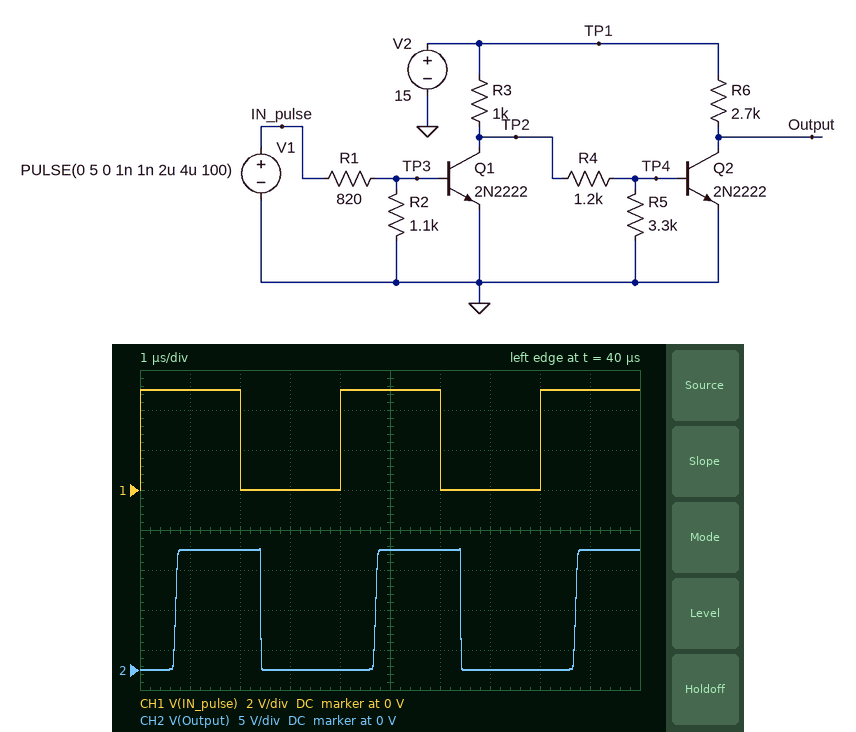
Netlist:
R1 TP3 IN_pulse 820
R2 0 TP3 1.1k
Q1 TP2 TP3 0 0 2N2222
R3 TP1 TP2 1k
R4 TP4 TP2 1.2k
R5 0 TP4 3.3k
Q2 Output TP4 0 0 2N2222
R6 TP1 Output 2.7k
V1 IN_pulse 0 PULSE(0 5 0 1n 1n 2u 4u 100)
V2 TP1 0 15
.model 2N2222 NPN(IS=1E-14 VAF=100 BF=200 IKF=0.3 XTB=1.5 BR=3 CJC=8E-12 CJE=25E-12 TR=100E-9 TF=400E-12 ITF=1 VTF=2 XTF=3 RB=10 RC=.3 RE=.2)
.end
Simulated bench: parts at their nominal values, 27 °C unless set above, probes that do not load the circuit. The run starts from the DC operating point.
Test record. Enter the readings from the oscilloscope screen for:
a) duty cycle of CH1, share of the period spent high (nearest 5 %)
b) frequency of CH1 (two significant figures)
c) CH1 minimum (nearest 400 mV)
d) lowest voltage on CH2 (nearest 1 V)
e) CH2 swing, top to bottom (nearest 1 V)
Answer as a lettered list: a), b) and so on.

a) 50 %
b) 250 kHz
c) 0 V
d) 0 V
e) 15 V
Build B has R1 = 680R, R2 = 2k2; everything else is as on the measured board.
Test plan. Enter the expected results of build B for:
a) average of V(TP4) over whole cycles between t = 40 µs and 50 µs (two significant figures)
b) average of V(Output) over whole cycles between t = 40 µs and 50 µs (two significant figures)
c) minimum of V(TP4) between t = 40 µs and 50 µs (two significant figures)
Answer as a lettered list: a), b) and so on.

a) 450 mV
b) 6.7 V
c) 19 mV
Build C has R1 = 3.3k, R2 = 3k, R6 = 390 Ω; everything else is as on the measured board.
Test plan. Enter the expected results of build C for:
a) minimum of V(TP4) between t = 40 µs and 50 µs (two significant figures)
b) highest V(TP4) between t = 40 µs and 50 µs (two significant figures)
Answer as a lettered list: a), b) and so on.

a) 42 mV
b) 840 mV
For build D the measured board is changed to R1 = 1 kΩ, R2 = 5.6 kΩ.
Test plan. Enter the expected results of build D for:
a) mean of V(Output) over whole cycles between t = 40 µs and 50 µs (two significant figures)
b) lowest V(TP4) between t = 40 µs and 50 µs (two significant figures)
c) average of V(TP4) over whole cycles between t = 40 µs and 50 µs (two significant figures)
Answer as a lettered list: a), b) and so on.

a) 6.8 V
b) 23 mV
c) 450 mV
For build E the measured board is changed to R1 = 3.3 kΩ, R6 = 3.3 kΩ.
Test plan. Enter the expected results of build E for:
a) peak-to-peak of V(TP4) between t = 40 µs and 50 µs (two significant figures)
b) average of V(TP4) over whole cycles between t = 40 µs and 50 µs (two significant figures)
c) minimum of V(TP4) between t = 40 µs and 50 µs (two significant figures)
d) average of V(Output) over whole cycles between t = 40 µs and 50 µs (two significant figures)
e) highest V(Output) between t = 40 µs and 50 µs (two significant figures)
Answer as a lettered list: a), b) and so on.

a) 760 mV
b) 540 mV
c) 51 mV
d) 5.2 V
e) 15 V
